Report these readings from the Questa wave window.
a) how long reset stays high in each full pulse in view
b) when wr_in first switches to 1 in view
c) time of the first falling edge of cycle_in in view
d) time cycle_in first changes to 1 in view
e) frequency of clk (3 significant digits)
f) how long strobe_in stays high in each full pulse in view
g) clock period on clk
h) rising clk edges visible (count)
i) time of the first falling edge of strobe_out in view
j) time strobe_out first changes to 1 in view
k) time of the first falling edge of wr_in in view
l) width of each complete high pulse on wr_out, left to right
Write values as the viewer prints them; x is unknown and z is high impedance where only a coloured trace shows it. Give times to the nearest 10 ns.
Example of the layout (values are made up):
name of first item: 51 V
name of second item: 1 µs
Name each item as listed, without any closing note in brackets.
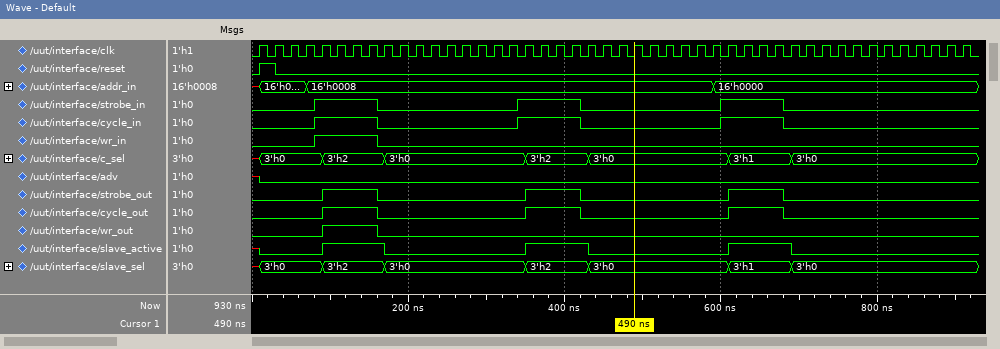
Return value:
how long reset stays high in each full pulse in view: 20 ns
when wr_in first switches to 1 in view: 80 ns
time of the first falling edge of cycle_in in view: 160 ns
time cycle_in first changes to 1 in view: 80 ns
frequency of clk: 50.0 MHz
how long strobe_in stays high in each full pulse in view: 80 ns, 80 ns, 80 ns
clock period on clk: 20 ns
rising clk edges visible: 46
time of the first falling edge of strobe_out in view: 160 ns
time strobe_out first changes to 1 in view: 90 ns
time of the first falling edge of wr_in in view: 160 ns
width of each complete high pulse on wr_out, left to right: 70 ns
